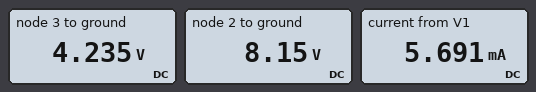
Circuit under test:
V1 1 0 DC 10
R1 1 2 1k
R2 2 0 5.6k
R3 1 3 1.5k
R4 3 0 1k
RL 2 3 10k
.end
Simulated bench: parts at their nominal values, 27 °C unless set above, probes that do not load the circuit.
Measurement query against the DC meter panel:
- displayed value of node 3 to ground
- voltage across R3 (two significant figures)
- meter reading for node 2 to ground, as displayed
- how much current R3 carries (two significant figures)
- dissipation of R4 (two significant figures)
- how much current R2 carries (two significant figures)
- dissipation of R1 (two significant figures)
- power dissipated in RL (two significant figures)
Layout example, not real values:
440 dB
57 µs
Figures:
4.235 V
5.8 V
8.15 V
3.8 mA
18 mW
1.5 mA
3.4 mW
1.5 mW
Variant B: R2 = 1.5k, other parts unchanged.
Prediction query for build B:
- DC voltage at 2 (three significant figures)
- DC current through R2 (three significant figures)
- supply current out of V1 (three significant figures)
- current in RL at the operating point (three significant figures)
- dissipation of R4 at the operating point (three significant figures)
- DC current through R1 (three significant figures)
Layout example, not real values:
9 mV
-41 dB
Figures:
5.89 V
3.93 mA
8.04 mA
179 µA
16.9 mW
4.11 mA
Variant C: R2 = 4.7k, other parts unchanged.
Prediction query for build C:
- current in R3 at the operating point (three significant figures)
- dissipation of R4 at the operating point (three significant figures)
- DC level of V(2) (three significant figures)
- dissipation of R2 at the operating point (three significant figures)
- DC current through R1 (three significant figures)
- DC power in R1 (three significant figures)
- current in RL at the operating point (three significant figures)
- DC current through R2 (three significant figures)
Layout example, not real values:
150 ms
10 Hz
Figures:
3.85 mA
17.8 mW
7.94 V
13.4 mW
2.06 mA
4.25 mW
372 µA
1.69 mA
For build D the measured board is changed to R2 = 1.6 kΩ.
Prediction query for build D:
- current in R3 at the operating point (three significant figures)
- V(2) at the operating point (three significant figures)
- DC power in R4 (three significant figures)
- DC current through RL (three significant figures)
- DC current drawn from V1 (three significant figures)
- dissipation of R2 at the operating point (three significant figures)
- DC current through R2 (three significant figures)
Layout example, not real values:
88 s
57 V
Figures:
3.92 mA
6.04 V
16.9 mW
192 µA
7.89 mA
22.8 mW
3.77 mA
